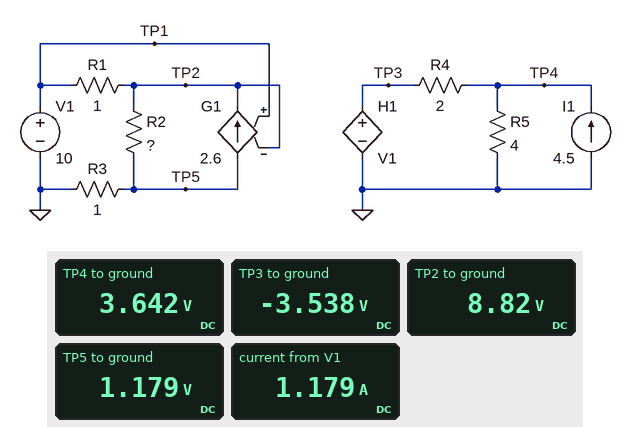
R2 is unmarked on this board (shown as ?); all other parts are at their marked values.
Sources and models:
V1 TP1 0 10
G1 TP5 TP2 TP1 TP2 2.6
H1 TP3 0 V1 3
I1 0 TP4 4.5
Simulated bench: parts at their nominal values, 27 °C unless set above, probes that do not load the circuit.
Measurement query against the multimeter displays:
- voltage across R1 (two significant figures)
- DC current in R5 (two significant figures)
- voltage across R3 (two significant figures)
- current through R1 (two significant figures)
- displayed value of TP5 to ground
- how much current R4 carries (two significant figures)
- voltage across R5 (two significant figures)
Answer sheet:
1.2 V
910 mA
1.2 V
1.2 A
1.179 V
3.6 A
3.6 V
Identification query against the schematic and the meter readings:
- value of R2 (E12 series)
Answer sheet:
1.8 Ω
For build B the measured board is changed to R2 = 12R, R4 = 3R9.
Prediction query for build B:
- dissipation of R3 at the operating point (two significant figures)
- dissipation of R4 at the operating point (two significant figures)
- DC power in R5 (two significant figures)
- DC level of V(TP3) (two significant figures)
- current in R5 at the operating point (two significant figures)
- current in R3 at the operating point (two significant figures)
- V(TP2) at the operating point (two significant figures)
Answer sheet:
49 mW
22 W
18 W
-660 mV
2.1 A
220 mA
9.8 V
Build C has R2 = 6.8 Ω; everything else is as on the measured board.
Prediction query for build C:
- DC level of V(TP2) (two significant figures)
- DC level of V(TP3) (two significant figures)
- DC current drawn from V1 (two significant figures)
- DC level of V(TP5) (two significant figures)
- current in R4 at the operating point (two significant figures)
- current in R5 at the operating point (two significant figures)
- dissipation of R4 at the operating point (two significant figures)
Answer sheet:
9.6 V
-1.1 V
380 mA
380 mV
3.2 A
1.3 A
20 W
